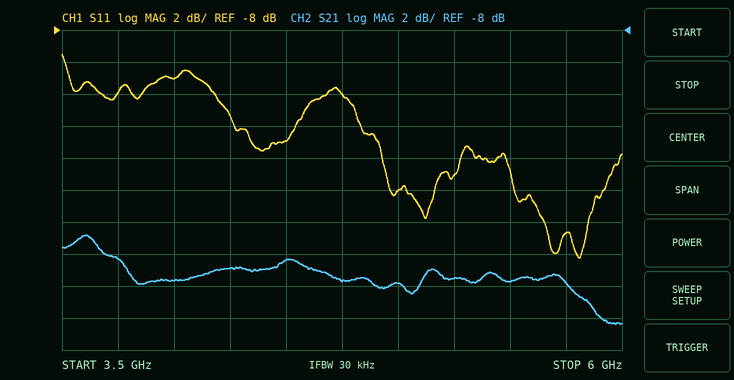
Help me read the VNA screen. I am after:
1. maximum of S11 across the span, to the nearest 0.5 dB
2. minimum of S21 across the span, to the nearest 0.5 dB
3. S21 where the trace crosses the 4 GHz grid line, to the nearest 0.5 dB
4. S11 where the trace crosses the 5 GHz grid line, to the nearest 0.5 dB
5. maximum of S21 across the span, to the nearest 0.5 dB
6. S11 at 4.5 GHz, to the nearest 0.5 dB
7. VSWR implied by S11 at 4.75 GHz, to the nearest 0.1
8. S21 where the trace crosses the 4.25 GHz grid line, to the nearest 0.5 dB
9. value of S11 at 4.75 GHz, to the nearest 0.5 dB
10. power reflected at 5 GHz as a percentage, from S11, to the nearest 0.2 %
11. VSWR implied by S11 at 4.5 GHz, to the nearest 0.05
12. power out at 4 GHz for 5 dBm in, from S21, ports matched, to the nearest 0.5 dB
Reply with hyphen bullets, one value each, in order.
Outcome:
- -9.5 dB
- -26.5 dB
- -23.5 dB
- -18.0 dB
- -21.0 dB
- -15.0 dB
- 1.7
- -23.0 dB
- -12.0 dB
- 1.6 %
- 1.45
- -18.5 dBm
